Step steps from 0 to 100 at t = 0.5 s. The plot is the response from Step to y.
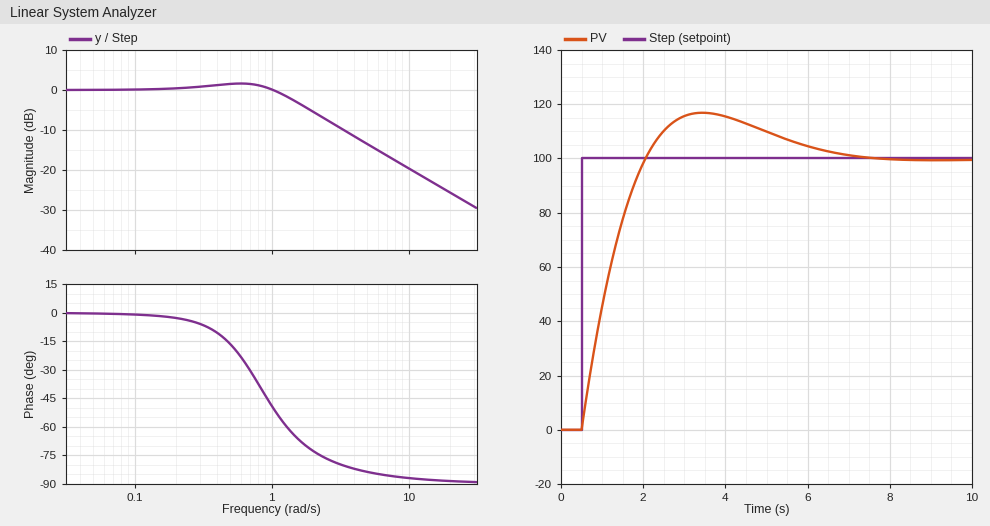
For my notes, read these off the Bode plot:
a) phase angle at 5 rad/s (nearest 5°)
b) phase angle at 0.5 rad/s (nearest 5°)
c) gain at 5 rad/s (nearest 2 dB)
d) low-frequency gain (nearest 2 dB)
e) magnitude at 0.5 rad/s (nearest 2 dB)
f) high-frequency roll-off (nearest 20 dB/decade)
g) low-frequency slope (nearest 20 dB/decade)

-85°
-15°
-14 dB
0 dB
2 dB
-20 dB/decade
0 dB/decade
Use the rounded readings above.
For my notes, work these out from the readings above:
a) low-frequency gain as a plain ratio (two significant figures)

1.0
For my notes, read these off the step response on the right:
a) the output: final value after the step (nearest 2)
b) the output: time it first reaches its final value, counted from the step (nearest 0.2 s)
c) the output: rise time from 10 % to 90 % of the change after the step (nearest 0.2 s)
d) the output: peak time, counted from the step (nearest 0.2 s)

100
1.6 s
1.2 s
3.0 s
